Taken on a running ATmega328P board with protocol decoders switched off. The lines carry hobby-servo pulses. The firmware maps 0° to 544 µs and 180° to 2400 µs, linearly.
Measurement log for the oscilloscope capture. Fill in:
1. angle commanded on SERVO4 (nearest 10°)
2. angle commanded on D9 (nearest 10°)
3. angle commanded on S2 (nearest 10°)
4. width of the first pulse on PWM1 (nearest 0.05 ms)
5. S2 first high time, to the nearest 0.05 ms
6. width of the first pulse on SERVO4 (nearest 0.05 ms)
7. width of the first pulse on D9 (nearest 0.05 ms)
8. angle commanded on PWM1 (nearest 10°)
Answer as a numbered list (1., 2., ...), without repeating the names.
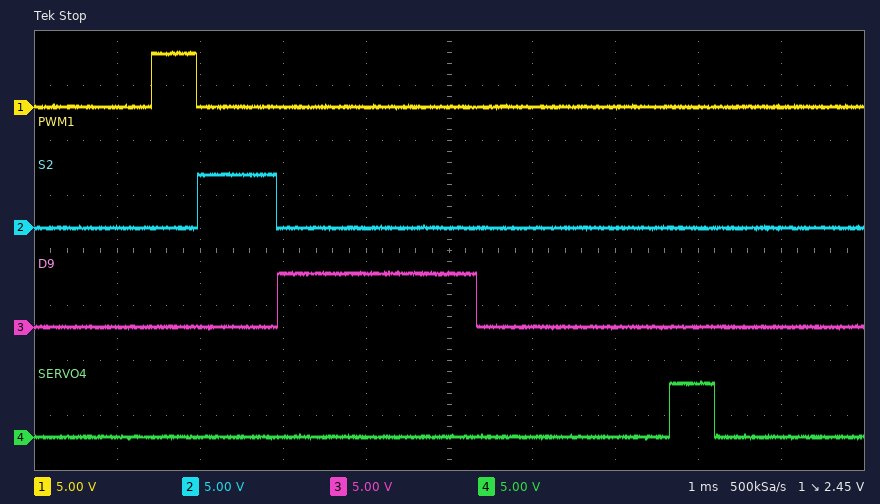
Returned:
1. 0°
2. 180°
3. 40°
4. 0.55 ms
5. 0.95 ms
6. 0.55 ms
7. 2.40 ms
8. 0°
